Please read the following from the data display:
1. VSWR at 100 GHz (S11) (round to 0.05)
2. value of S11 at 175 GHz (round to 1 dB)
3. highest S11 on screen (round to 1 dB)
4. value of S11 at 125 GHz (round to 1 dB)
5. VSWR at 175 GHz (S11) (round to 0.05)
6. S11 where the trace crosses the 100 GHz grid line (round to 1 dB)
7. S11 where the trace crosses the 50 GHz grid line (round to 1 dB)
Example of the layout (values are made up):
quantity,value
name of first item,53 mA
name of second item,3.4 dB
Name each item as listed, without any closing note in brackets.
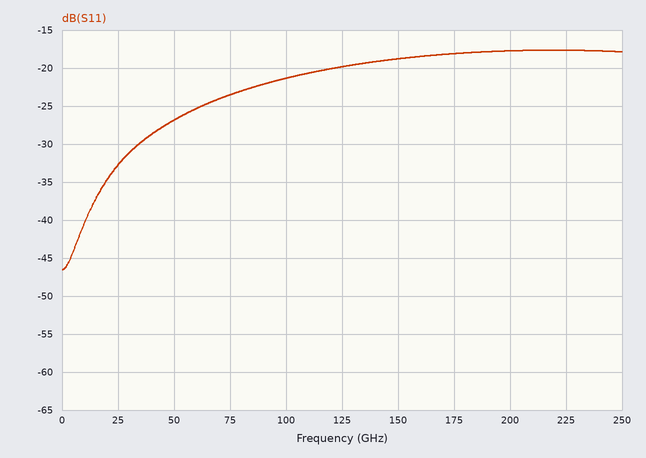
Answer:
quantity,value
VSWR at 100 GHz (S11),1.20
value of S11 at 175 GHz,-18 dB
highest S11 on screen,-18 dB
value of S11 at 125 GHz,-20 dB
VSWR at 175 GHz (S11),1.30
S11 where the trace crosses the 100 GHz grid line,-21 dB
S11 where the trace crosses the 50 GHz grid line,-27 dB
